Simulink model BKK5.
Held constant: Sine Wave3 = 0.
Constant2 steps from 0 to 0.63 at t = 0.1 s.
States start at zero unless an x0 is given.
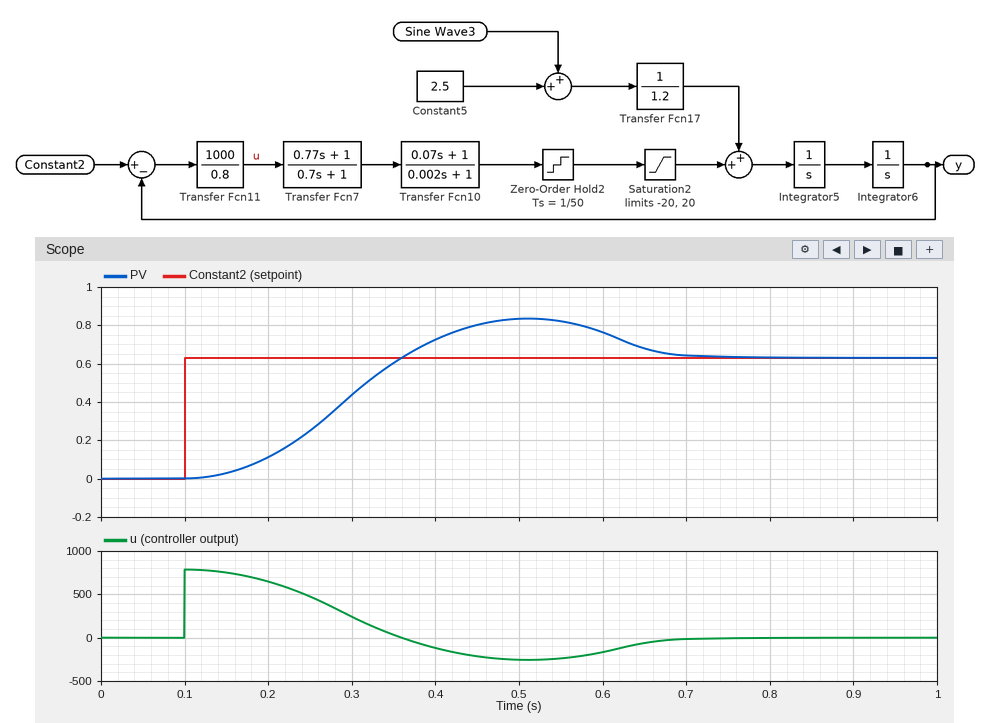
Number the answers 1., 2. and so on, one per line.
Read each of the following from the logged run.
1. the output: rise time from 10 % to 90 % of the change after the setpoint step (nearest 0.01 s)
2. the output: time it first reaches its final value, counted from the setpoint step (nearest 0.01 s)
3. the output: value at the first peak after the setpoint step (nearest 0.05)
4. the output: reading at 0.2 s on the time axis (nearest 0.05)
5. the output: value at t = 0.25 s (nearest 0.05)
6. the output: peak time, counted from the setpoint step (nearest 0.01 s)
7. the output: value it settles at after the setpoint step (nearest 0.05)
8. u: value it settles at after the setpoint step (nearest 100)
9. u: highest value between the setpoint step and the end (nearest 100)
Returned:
1. 0.16 s
2. 0.26 s
3. 0.85
4. 0.10
5. 0.25
6. 0.41 s
7. 0.65
8. 0
9. 800
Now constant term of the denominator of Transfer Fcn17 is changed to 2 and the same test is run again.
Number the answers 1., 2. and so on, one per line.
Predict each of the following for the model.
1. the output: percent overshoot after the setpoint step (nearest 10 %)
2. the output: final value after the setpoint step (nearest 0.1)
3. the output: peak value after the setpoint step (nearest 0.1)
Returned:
1. 40 %
2. 0.6
3. 0.9
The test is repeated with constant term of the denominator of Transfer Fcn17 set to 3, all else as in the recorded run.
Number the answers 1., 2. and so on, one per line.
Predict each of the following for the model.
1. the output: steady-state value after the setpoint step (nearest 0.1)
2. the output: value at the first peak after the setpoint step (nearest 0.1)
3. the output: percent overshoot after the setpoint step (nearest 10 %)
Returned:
1. 0.6
2. 0.9
3. 40 %
